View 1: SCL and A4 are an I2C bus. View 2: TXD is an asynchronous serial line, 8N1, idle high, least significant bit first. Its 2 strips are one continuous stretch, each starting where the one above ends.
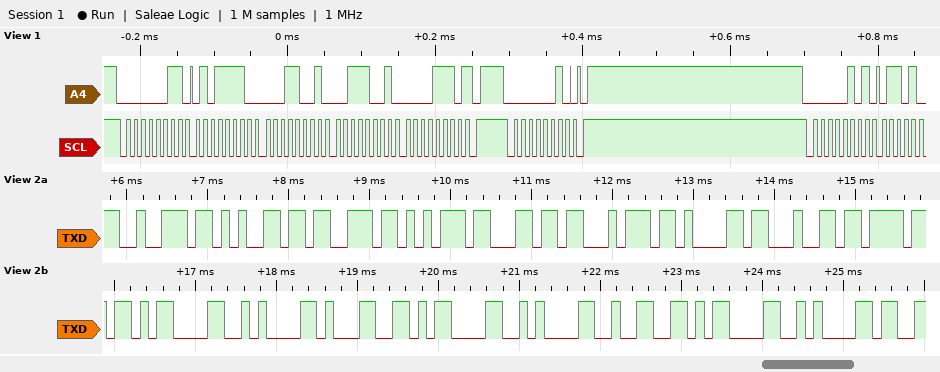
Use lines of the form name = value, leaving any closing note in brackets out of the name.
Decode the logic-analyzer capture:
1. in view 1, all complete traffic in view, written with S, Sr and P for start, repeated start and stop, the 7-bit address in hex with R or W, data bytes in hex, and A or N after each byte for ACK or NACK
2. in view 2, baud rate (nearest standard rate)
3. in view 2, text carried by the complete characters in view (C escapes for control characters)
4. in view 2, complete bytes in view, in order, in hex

in view 1, all complete traffic in view, written with S, Sr and P for start, repeated start and stop, the 7-bit address in hex with R or W, data bytes in hex, and A or N after each byte for ACK or NACK = S 01R A 5E A 19 A 39 A 0E N P S 01W A P S 02R A
in view 2, baud rate = 9600 baud
in view 2, text carried by the complete characters in view = "resultado\r\n1\r\n2\r\n"
in view 2, complete bytes in view, in order, in hex = 72 65 73 75 6C 74 61 64 6F 0D 0A 31 0D 0A 32 0D 0A
